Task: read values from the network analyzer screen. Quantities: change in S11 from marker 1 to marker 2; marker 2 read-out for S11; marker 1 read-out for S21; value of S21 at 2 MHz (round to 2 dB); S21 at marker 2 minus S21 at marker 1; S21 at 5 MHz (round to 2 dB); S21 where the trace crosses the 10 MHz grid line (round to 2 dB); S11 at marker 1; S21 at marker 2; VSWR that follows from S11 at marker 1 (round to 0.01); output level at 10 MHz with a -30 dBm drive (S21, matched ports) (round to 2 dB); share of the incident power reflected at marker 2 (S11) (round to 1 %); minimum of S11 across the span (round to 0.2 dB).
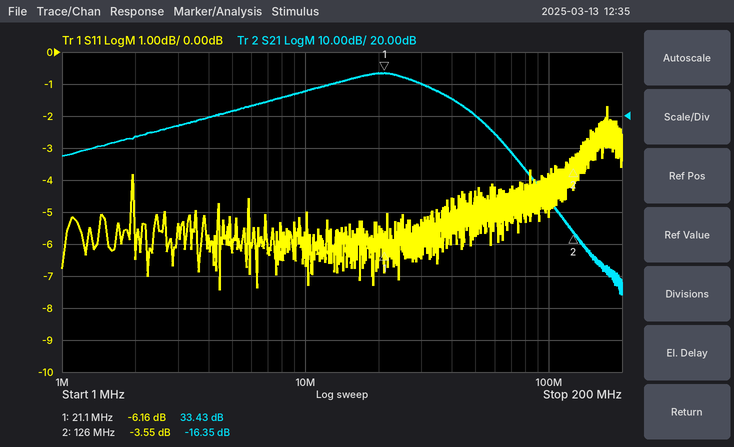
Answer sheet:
2.61 dB
-3.55 dB
33.43 dB
14 dB
-49.78 dB
22 dB
28 dB
-6.16 dB
-16.35 dB
2.94
-2 dBm
44 %
-7.4 dB
